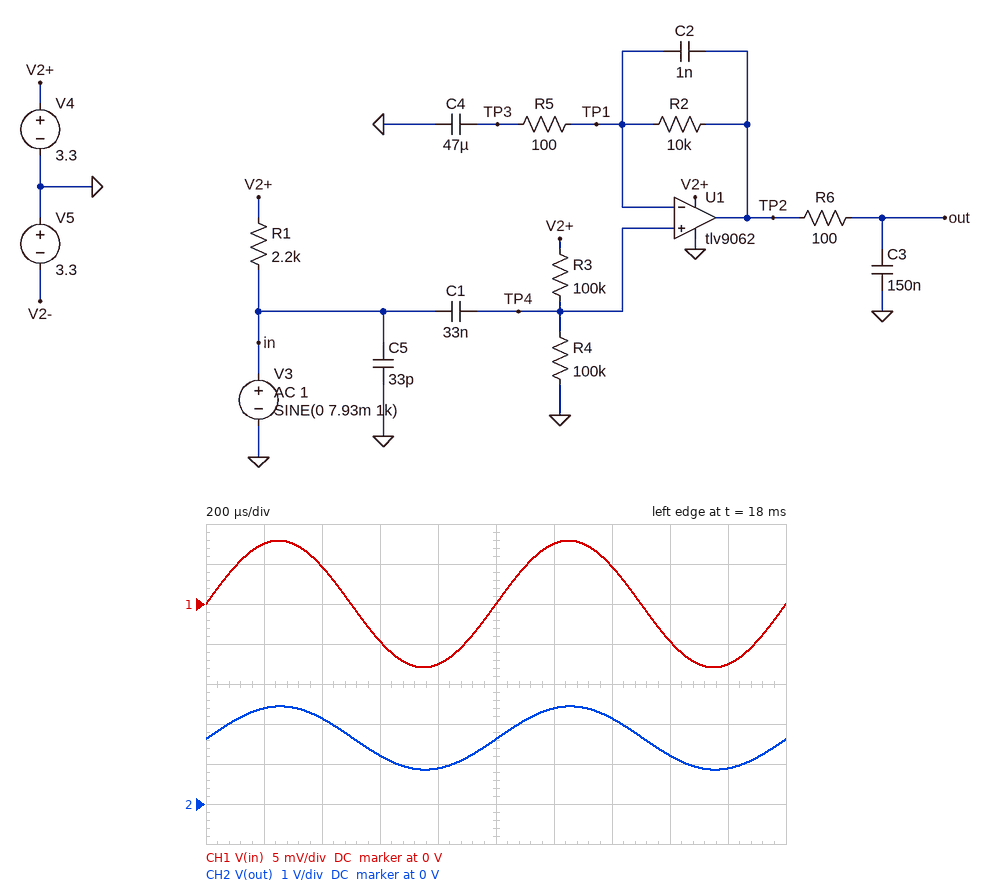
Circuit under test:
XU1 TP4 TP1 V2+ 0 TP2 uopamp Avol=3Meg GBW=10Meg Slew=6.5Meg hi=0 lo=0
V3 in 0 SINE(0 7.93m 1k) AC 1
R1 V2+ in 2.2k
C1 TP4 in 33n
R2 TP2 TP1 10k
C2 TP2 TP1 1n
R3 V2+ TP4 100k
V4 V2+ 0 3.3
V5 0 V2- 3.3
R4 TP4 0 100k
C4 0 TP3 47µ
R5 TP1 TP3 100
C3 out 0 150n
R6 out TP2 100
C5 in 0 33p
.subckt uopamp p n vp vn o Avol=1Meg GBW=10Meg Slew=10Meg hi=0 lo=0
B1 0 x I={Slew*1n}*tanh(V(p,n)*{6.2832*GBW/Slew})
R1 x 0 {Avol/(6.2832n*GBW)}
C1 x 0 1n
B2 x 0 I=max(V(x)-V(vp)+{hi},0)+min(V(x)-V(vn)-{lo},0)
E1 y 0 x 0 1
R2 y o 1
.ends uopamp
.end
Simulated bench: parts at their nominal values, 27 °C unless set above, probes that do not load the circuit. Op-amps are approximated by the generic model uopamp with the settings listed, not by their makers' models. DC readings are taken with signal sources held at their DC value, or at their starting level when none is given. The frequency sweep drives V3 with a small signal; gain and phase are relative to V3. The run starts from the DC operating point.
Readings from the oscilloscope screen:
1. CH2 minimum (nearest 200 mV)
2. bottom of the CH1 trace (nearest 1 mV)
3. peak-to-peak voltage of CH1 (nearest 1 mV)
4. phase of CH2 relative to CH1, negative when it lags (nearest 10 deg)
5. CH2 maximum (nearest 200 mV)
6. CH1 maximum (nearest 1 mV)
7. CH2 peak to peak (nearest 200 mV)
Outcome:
800 mV
-8 mV
16 mV
0 deg
2.4 V
8 mV
1.6 V
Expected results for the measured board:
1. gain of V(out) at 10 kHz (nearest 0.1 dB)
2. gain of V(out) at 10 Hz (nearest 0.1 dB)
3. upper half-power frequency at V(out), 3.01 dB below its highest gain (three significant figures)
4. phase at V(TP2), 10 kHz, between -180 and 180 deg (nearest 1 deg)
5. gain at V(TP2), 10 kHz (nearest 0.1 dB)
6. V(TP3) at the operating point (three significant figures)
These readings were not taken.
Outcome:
35.5 dB
9.4 dB
7.84 kHz
-35 deg
38.2 dB
1.65 V
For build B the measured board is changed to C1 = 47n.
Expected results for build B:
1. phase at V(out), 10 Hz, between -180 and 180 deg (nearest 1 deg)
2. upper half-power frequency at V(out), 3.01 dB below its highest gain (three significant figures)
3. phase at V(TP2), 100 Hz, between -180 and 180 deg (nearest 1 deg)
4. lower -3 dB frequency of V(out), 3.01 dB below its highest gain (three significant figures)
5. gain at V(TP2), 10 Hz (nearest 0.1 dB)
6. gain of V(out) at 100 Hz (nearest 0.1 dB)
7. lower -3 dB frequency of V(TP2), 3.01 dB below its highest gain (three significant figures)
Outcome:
153 deg
7.80 kHz
52 deg
79.6 Hz
12.4 dB
38.0 dB
80.1 Hz
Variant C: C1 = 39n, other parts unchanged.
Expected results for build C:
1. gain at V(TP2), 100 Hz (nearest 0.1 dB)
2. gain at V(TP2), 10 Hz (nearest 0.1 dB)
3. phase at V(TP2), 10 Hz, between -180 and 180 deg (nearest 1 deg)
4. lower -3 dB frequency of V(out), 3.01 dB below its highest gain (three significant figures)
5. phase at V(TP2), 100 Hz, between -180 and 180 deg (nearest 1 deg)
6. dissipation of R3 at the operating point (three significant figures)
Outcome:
37.4 dB
10.8 dB
155 deg
91.5 Hz
57 deg
27.2 µW
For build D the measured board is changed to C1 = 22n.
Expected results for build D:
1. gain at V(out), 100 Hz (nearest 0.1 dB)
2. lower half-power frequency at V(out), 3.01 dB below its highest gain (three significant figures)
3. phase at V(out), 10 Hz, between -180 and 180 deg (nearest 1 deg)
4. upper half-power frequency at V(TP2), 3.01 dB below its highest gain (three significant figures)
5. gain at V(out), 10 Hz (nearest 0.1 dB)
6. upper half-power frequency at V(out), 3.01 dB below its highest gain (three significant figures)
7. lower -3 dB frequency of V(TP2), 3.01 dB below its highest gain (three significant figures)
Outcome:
34.7 dB
147 Hz
158 deg
14.0 kHz
5.9 dB
7.91 kHz
149 Hz
